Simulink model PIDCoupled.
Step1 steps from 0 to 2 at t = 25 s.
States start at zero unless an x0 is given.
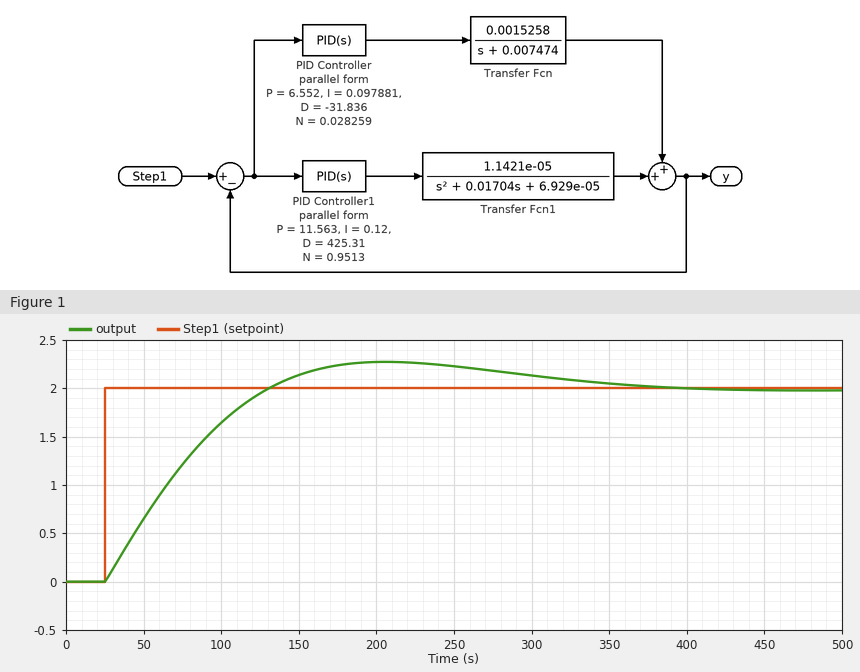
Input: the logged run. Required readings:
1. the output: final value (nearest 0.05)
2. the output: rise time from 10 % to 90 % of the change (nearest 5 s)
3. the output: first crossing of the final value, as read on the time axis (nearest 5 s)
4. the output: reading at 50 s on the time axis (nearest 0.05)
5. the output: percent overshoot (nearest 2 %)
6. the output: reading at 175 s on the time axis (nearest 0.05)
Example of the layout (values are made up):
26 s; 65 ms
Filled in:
2.00; 80 s; 130 s; 0.65; 14 %; 2.25
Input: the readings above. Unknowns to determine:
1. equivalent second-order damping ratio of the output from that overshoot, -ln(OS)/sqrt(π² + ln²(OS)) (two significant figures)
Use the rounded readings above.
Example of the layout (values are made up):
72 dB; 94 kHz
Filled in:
0.53
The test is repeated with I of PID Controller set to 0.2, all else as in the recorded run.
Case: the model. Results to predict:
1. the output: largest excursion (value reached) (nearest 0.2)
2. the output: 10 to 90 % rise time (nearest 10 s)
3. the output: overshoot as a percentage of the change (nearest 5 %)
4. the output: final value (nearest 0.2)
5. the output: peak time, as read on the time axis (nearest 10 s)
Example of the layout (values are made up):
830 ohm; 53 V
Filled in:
2.4; 60 s; 20 %; 2.0; 160 s
